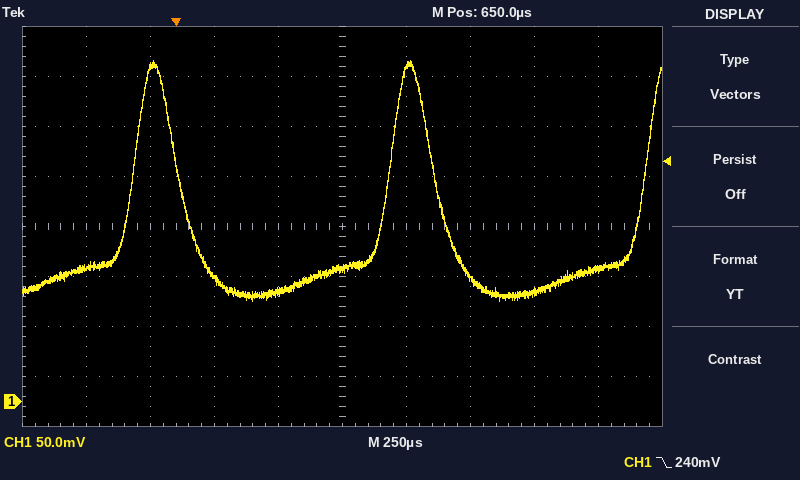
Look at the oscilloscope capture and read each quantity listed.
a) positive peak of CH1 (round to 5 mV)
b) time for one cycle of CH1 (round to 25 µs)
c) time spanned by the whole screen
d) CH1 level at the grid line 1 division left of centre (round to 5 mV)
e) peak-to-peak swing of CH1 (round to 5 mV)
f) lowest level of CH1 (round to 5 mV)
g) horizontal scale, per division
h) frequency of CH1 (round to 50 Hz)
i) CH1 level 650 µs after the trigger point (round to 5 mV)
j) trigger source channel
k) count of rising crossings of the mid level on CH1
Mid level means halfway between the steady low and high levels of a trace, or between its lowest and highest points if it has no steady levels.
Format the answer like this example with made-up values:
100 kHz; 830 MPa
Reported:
340 mV; 1.000 ms; 2.5 ms; 110 mV; 240 mV; 100 mV; 250 µs; 1.00 kHz; 135 mV; CH1; 3
